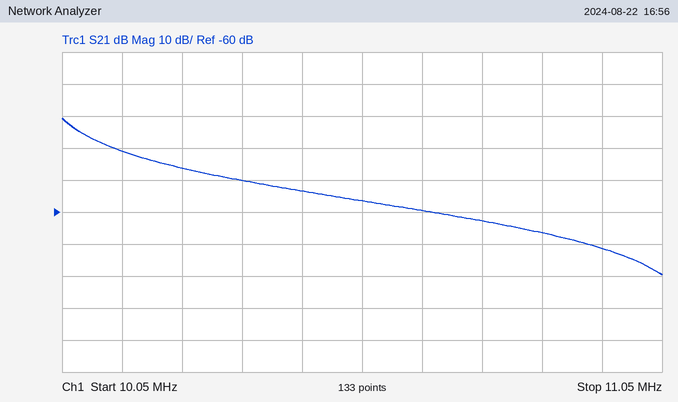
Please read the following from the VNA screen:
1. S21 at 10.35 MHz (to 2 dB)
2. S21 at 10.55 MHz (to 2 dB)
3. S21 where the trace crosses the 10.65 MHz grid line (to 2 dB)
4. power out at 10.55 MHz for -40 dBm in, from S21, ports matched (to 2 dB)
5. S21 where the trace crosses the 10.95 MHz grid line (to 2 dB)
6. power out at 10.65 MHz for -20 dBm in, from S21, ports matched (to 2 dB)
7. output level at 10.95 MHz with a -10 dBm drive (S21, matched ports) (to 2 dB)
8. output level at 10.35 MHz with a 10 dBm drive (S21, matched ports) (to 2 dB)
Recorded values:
-50 dB
-56 dB
-60 dB
-96 dBm
-72 dB
-80 dBm
-82 dBm
-40 dBm
